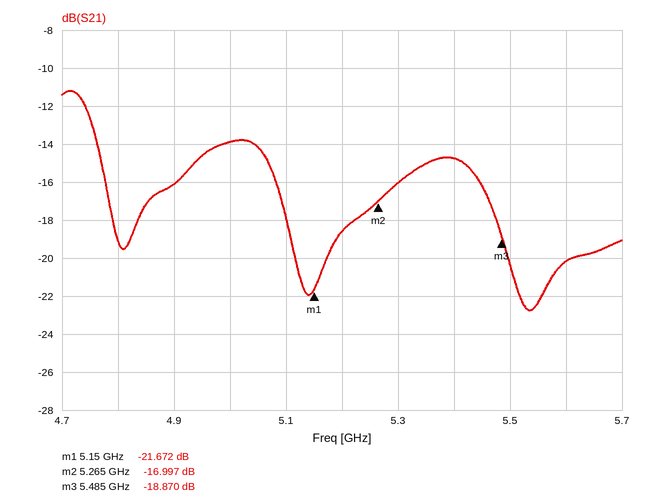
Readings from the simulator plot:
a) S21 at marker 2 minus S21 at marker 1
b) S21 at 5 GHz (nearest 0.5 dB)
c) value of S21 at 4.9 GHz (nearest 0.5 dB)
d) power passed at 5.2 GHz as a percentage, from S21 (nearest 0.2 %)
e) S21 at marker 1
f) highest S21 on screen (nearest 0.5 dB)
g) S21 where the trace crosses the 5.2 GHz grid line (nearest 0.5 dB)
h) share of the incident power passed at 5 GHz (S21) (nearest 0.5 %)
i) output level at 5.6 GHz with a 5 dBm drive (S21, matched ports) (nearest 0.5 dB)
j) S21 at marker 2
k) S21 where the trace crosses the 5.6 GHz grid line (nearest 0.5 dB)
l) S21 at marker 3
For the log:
4.675 dB
-14.0 dB
-16.0 dB
1.4 %
-21.672 dB
-11.0 dB
-18.5 dB
4.0 %
-15.0 dBm
-16.997 dB
-20.0 dB
-18.870 dB
